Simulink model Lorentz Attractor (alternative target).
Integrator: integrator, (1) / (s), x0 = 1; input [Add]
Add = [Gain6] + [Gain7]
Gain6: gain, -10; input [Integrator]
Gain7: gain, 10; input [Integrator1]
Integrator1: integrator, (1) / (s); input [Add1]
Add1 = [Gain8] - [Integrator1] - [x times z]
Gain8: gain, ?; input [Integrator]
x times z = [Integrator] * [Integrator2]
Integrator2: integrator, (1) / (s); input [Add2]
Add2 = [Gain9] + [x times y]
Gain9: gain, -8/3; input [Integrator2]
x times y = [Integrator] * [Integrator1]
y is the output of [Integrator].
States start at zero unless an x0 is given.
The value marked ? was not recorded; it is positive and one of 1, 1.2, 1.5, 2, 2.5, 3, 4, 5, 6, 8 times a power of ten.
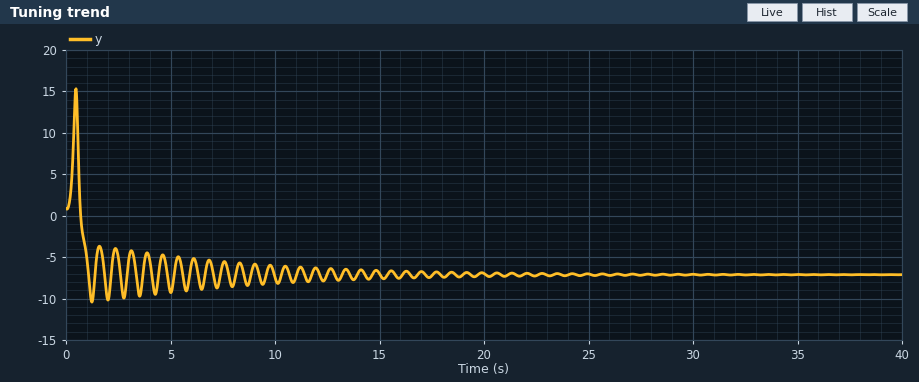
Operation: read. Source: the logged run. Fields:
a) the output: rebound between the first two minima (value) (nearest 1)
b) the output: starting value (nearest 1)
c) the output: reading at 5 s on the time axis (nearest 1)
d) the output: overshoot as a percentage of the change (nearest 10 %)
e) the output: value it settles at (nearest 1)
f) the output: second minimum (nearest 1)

-4
1
-9
40 %
-7
-10
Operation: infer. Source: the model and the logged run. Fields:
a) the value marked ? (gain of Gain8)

20
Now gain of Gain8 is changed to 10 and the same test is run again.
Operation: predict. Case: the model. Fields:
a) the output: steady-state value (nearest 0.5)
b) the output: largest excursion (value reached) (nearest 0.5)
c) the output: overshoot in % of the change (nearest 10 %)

5.0
8.5
100 %
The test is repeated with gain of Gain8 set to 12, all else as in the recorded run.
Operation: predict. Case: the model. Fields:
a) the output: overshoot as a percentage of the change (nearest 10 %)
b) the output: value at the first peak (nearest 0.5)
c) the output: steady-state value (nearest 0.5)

110 %
10.0
5.5
